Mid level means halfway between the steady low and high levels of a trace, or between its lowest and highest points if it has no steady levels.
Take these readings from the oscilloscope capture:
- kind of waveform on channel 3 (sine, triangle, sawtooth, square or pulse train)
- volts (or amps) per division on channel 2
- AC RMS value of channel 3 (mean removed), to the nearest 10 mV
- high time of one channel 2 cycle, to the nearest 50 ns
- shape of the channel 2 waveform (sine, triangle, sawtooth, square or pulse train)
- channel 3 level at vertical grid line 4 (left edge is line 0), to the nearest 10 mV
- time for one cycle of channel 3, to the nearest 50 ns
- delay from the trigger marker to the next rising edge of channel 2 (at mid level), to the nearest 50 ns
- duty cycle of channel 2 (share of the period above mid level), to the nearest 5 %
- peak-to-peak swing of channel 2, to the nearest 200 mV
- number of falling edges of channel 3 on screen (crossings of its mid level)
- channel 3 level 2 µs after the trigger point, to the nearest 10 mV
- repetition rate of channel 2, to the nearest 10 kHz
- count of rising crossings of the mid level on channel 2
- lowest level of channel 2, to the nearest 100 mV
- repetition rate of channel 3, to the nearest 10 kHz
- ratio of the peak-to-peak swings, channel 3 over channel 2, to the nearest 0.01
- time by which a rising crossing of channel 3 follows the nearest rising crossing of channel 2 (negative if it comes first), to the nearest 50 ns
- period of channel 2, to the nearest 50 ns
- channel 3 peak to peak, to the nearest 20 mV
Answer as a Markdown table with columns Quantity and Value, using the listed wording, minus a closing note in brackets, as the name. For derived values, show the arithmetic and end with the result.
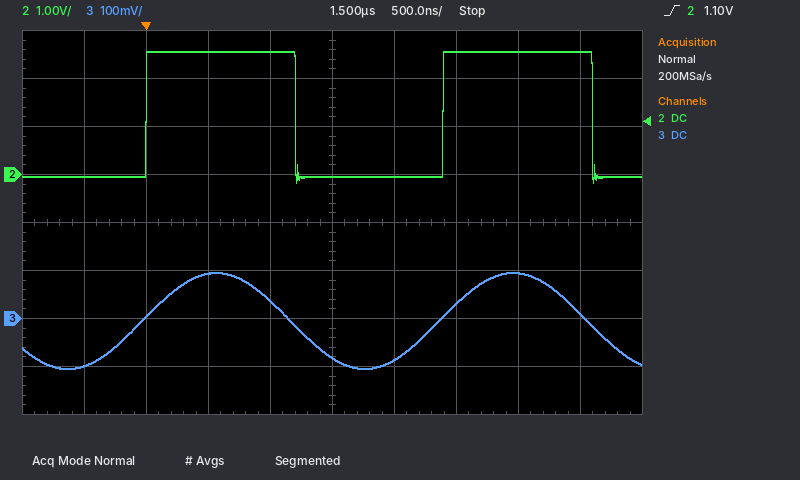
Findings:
| Quantity | Value |
|---|---|
| kind of waveform on channel 3 | sine |
| volts (or amps) per division on channel 2 | 1 V |
| AC RMS value of channel 3 (mean removed), to the nearest 10 mV | 200 mV / (2√2) ≈ 70.7 mV, so 70 mV to the nearest 10 mV |
| high time of one channel 2 cycle, to the nearest 50 ns | 1.20 µs |
| shape of the channel 2 waveform | square |
| channel 3 level at vertical grid line 4 (left edge is line 0), to the nearest 10 mV | 40 mV |
| time for one cycle of channel 3, to the nearest 50 ns | 2.40 µs |
| delay from the trigger marker to the next rising edge of channel 2 (at mid level), to the nearest 50 ns | 2.40 µs |
| duty cycle of channel 2 (share of the period above mid level), to the nearest 5 % | 1.20 µs / 2.40 µs ≈ 50 % |
| peak-to-peak swing of channel 2, to the nearest 200 mV | 2.8 V |
| number of falling edges of channel 3 on screen | 2 |
| channel 3 level 2 µs after the trigger point, to the nearest 10 mV | -90 mV |
| repetition rate of channel 2, to the nearest 10 kHz | 1 / 2.40 µs ≈ 417 kHz, so 420 kHz to the nearest 10 kHz |
| count of rising crossings of the mid level on channel 2 | 2 |
| lowest level of channel 2, to the nearest 100 mV | -200 mV |
| repetition rate of channel 3, to the nearest 10 kHz | 1 / 2.40 µs ≈ 417 kHz, so 420 kHz to the nearest 10 kHz |
| ratio of the peak-to-peak swings, channel 3 over channel 2, to the nearest 0.01 | 200 mV / 2.8 V ≈ 0.07 |
| time by which a rising crossing of channel 3 follows the nearest rising crossing of channel 2 (negative if it comes first), to the nearest 50 ns | -50 ns |
| period of channel 2, to the nearest 50 ns | 2.40 µs |
| channel 3 peak to peak, to the nearest 20 mV | 200 mV |
